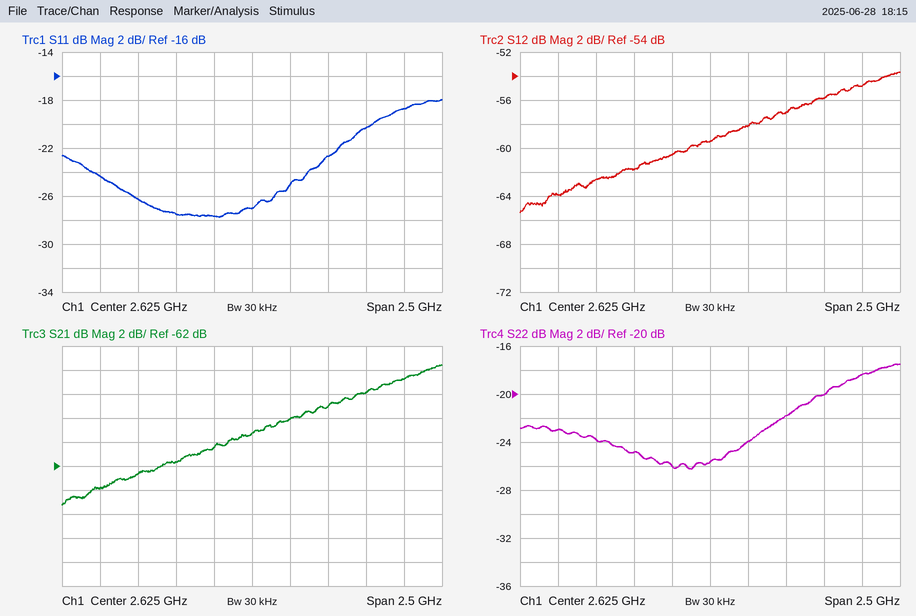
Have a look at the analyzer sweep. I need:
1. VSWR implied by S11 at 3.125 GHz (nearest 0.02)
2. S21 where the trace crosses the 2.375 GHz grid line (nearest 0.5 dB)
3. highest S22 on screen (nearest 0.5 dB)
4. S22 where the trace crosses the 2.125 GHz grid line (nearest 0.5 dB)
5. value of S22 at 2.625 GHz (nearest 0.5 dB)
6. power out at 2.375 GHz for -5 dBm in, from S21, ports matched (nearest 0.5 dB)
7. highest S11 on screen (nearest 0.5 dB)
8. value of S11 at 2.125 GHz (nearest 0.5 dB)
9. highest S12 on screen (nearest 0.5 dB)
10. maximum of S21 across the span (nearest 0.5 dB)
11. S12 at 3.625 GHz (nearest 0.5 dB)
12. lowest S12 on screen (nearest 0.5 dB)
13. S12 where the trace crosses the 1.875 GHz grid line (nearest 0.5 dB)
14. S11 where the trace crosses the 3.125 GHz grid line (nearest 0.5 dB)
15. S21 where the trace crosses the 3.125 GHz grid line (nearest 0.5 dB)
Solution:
1.16
-60.5 dB
-17.5 dB
-25.0 dB
-25.5 dB
-65.5 dBm
-18.0 dB
-27.5 dB
-53.5 dB
-53.5 dB
-55.0 dB
-65.5 dB
-62.5 dB
-22.5 dB
-57.0 dB
